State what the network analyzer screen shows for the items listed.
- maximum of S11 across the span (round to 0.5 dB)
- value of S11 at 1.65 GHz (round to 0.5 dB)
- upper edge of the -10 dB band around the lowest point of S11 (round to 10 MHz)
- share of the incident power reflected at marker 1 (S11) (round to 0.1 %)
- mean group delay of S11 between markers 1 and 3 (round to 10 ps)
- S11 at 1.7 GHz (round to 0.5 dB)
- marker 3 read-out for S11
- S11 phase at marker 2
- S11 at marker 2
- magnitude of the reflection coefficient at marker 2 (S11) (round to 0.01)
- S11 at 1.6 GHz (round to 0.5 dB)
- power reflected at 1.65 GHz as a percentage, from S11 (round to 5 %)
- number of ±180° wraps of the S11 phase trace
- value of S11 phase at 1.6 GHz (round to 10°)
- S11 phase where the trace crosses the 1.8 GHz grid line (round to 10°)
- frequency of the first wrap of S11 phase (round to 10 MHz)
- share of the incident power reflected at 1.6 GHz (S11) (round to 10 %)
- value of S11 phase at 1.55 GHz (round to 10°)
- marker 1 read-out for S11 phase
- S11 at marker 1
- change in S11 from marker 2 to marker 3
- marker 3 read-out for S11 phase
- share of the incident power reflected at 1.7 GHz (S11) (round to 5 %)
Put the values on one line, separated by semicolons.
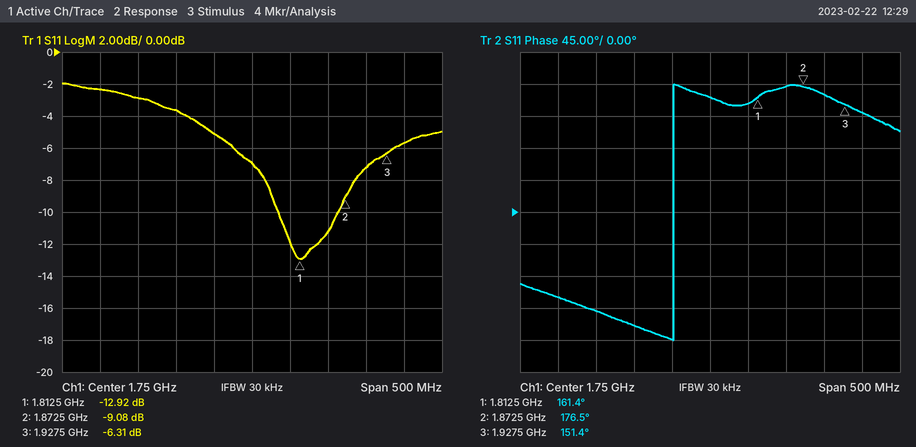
-2.0 dB; -3.5 dB; 1.86 GHz; 5.1 %; 240 ps; -5.0 dB; -6.31 dB; 176.5°; -9.08 dB; 0.35; -3.0 dB; 45 %; 1; -140°; 150°; 1.70 GHz; 50 %; -120°; 161.4°; -12.92 dB; 2.77 dB; 151.4°; 30 %
